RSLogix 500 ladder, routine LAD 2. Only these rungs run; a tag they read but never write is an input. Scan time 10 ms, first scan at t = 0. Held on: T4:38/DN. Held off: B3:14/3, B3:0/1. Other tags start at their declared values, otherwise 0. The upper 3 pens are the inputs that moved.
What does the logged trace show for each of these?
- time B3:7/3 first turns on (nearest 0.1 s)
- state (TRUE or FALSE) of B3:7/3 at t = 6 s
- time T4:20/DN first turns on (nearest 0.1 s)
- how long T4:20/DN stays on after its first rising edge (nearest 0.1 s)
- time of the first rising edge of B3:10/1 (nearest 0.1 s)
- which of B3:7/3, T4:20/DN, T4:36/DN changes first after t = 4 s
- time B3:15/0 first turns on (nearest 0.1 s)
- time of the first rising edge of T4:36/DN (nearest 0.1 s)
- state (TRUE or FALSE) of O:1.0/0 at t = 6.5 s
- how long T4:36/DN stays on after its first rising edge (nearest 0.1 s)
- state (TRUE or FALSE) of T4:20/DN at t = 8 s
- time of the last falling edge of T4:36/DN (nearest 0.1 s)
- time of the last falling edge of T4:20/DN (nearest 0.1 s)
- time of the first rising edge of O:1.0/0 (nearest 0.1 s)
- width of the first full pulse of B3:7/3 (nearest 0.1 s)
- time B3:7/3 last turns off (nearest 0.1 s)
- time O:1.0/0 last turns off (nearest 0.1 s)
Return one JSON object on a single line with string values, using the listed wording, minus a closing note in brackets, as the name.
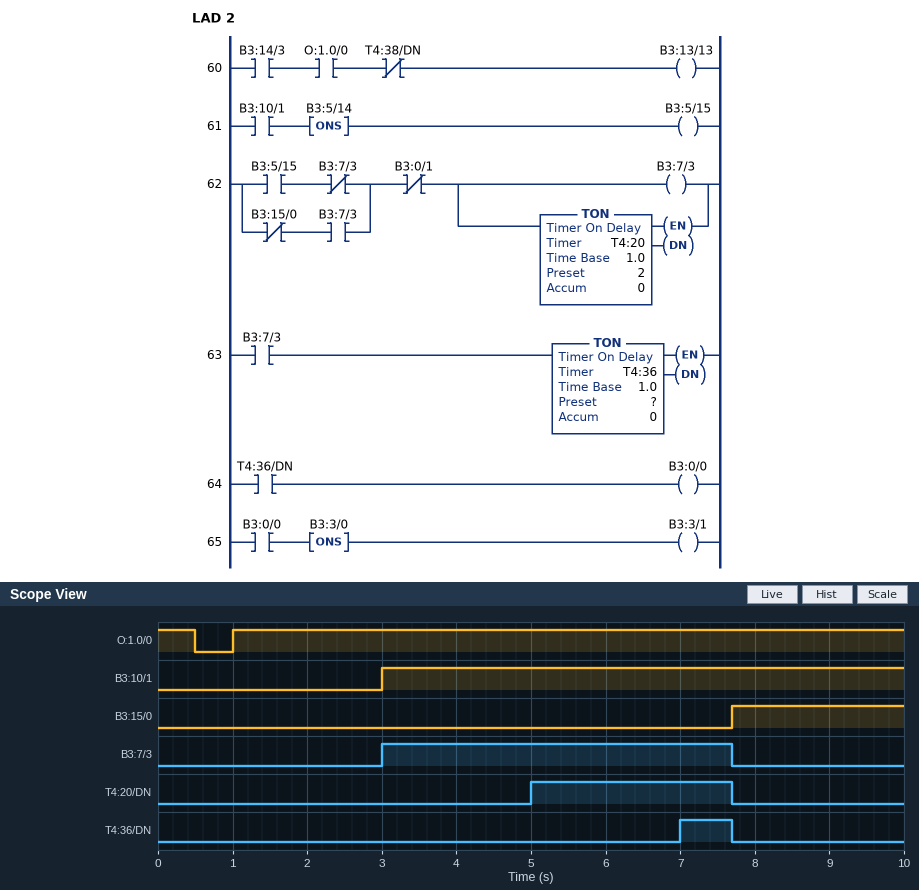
{"time B3:7/3 first turns on": "3.0 s", "state (TRUE or FALSE) of B3:7/3 at t = 6 s": "TRUE", "time T4:20/DN first turns on": "5.0 s", "how long T4:20/DN stays on after its first rising edge": "2.7 s", "time of the first rising edge of B3:10/1": "3.0 s", "which of B3:7/3, T4:20/DN, T4:36/DN changes first after t = 4 s": "T4:20/DN", "time B3:15/0 first turns on": "7.7 s", "time of the first rising edge of T4:36/DN": "7.0 s", "state (TRUE or FALSE) of O:1.0/0 at t = 6.5 s": "TRUE", "how long T4:36/DN stays on after its first rising edge": "0.7 s", "state (TRUE or FALSE) of T4:20/DN at t = 8 s": "FALSE", "time of the last falling edge of T4:36/DN": "7.7 s", "time of the last falling edge of T4:20/DN": "7.7 s", "time of the first rising edge of O:1.0/0": "1.0 s", "width of the first full pulse of B3:7/3": "4.7 s", "time B3:7/3 last turns off": "7.7 s", "time O:1.0/0 last turns off": "0.5 s"}
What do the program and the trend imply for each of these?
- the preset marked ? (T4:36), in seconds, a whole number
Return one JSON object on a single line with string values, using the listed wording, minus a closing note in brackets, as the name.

{"the preset marked ? (T4:36), in seconds, a whole number": "4 s"}
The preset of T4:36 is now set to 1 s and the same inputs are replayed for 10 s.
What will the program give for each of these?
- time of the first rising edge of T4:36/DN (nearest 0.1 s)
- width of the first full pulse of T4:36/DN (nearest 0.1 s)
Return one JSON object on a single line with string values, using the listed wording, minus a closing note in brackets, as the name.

{"time of the first rising edge of T4:36/DN": "4.0 s", "width of the first full pulse of T4:36/DN": "3.7 s"}
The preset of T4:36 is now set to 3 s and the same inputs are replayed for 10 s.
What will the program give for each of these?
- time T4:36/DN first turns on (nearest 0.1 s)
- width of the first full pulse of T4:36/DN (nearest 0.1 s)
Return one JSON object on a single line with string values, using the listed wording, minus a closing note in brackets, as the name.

{"time T4:36/DN first turns on": "6.0 s", "width of the first full pulse of T4:36/DN": "1.7 s"}
